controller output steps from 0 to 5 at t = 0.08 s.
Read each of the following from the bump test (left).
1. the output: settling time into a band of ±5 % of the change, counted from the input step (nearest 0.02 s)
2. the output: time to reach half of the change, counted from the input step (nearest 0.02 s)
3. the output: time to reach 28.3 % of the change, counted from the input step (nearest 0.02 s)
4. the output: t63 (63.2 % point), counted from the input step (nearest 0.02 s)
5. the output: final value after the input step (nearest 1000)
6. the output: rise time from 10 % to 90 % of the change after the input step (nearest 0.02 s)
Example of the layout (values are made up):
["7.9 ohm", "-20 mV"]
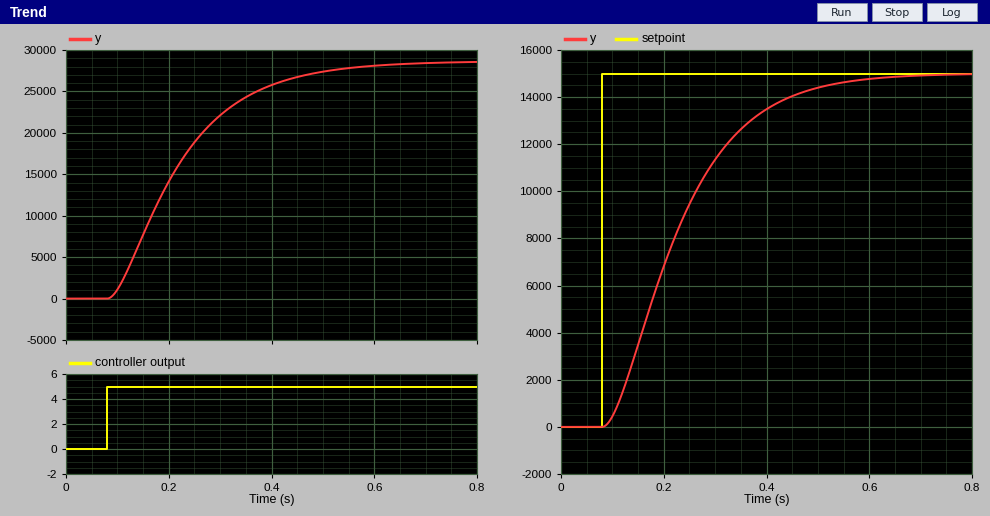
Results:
["0.40 s", "0.12 s", "0.08 s", "0.16 s", "29000", "0.28 s"]
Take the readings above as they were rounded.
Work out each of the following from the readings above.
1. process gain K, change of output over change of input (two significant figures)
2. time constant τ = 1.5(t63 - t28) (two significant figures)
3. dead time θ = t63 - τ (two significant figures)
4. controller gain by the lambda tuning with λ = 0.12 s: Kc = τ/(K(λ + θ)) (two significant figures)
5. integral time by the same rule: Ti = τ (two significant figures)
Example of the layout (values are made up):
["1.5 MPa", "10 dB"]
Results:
["5800", "0.12 s", "0.040 s", "0.00013", "0.12 s"]
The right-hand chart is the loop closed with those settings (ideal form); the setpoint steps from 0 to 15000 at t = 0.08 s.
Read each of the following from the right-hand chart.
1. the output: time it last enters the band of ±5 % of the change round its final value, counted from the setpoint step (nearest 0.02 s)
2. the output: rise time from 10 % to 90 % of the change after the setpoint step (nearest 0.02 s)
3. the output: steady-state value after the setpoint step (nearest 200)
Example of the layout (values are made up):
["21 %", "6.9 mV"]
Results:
["0.40 s", "0.28 s", "15000"]
